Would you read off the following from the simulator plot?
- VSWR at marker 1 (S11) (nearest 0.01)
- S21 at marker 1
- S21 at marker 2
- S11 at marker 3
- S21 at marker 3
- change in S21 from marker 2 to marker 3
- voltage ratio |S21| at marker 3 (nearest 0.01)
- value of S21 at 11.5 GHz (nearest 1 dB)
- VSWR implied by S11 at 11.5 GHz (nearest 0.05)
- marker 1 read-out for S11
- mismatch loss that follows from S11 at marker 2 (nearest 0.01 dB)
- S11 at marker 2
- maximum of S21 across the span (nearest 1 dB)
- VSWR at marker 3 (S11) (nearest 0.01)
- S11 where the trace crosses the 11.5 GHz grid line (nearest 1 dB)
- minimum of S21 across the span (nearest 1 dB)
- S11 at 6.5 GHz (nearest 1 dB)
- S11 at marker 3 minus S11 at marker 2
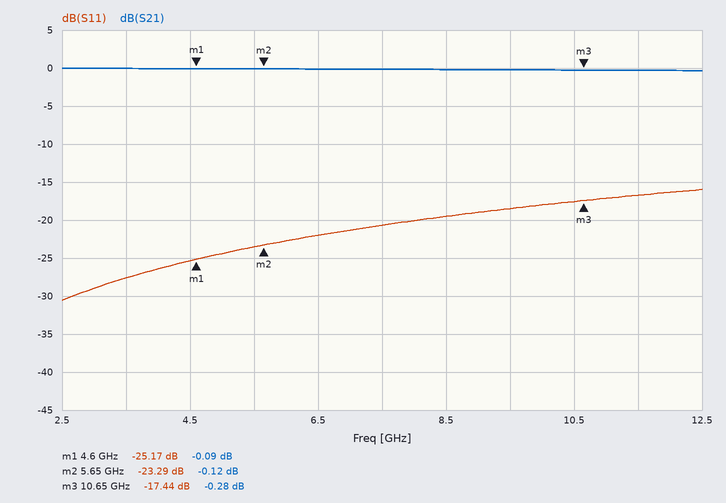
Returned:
1.12
-0.09 dB
-0.12 dB
-17.44 dB
-0.28 dB
-0.16 dB
0.97
0 dB
1.35
-25.17 dB
0.02 dB
-23.29 dB
0 dB
1.31
-17 dB
0 dB
-22 dB
5.85 dB
